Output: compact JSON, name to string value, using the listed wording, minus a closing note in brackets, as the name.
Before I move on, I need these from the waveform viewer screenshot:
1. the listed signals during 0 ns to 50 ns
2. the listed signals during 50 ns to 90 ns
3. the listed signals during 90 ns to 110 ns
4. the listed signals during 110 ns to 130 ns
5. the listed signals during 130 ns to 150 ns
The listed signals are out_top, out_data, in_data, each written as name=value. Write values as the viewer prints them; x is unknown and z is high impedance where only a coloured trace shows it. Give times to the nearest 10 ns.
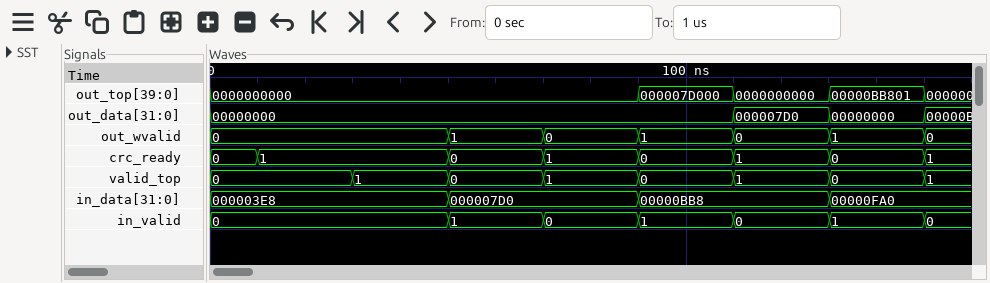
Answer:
{"the listed signals during 0 ns to 50 ns": "out_top=0000000000, out_data=00000000, in_data=000003E8", "the listed signals during 50 ns to 90 ns": "out_top=0000000000, out_data=00000000, in_data=000007D0", "the listed signals during 90 ns to 110 ns": "out_top=000007D000, out_data=00000000, in_data=00000BB8", "the listed signals during 110 ns to 130 ns": "out_top=0000000000, out_data=000007D0, in_data=00000BB8", "the listed signals during 130 ns to 150 ns": "out_top=00000BB801, out_data=00000000, in_data=00000FA0"}
